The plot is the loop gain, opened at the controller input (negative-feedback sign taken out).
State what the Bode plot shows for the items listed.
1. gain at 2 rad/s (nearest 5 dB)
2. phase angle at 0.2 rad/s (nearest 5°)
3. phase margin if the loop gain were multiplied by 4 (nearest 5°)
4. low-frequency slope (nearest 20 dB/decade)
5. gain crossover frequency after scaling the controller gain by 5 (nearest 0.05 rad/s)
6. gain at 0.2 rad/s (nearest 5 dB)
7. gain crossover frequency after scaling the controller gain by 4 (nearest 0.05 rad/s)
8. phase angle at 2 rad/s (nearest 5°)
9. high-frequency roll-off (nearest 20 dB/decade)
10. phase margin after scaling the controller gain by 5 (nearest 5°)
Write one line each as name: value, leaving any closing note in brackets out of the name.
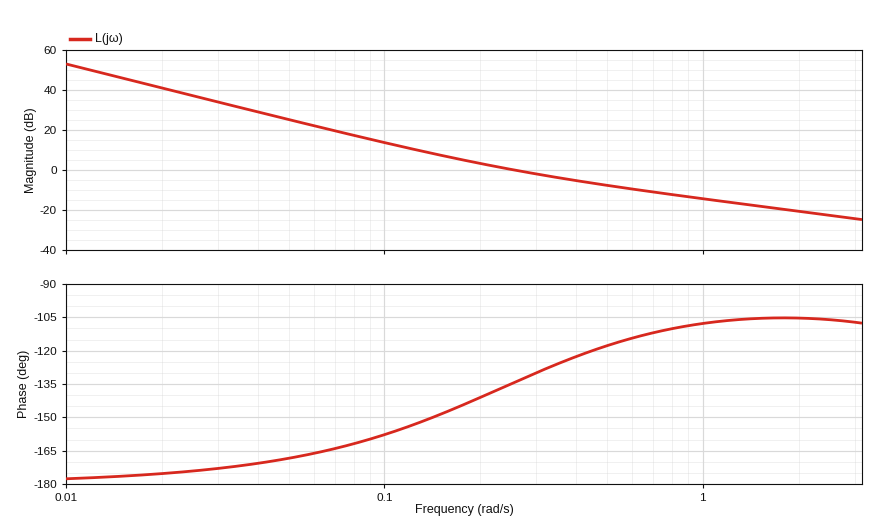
gain at 2 rad/s: -20 dB
phase angle at 0.2 rad/s: -140°
phase margin if the loop gain were multiplied by 4: 70°
low-frequency slope: -40 dB/decade
gain crossover frequency after scaling the controller gain by 5: 0.95 rad/s
gain at 0.2 rad/s: 5 dB
gain crossover frequency after scaling the controller gain by 4: 0.80 rad/s
phase angle at 2 rad/s: -105°
high-frequency roll-off: -20 dB/decade
phase margin after scaling the controller gain by 5: 70°
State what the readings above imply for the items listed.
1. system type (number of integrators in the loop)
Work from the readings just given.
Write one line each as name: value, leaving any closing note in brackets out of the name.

system type: 2
